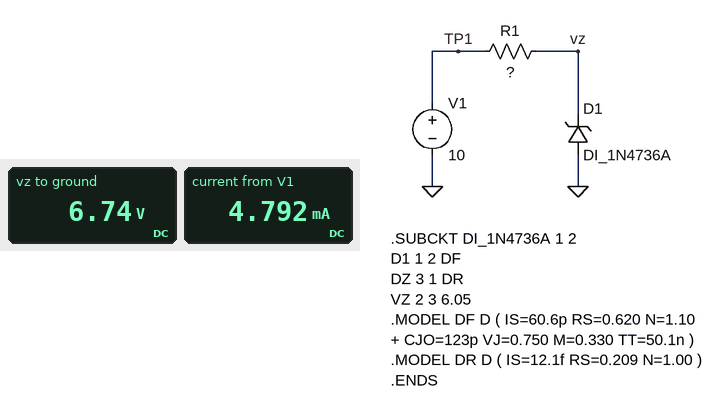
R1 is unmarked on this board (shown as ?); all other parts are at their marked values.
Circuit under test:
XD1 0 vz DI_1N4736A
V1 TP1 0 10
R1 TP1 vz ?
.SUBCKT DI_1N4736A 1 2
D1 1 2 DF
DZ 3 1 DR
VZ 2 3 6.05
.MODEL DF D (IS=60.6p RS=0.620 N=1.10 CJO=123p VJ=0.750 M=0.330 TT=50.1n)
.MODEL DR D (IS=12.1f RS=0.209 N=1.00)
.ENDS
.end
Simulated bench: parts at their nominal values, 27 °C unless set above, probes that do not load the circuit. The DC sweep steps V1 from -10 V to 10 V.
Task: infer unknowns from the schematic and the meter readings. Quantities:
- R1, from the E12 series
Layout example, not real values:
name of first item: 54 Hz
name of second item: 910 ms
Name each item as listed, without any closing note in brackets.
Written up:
R1, from the E12 series: 680 Ω
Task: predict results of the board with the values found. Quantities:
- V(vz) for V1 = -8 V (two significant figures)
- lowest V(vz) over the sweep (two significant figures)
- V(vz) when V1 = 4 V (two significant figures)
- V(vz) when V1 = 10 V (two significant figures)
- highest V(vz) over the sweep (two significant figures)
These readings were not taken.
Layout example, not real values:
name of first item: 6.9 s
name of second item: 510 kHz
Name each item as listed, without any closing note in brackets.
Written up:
V(vz) for V1 = -8 V: -550 mV
lowest V(vz) over the sweep: -560 mV
V(vz) when V1 = 4 V: 4.0 V
V(vz) when V1 = 10 V: 6.7 V
highest V(vz) over the sweep: 6.7 V
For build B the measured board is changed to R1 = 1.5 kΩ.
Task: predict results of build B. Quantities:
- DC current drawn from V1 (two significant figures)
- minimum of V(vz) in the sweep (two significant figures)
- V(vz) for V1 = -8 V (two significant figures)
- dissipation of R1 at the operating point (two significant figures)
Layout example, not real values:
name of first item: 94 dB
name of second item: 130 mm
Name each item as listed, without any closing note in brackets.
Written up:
DC current drawn from V1: 2.2 mA
minimum of V(vz) in the sweep: -530 mV
V(vz) for V1 = -8 V: -520 mV
dissipation of R1 at the operating point: 7.2 mW
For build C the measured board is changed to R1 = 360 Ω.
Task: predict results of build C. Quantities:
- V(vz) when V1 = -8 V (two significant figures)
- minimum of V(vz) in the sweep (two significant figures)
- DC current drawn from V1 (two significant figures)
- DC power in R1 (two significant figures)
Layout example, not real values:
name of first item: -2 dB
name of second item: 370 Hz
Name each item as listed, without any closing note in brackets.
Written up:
V(vz) when V1 = -8 V: -570 mV
minimum of V(vz) in the sweep: -580 mV
DC current drawn from V1: 9.0 mA
DC power in R1: 29 mW
